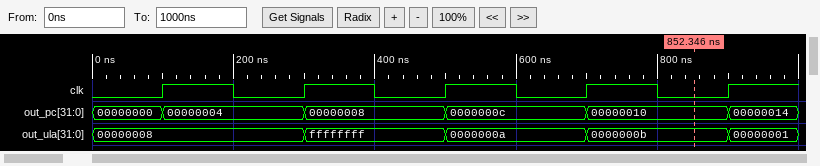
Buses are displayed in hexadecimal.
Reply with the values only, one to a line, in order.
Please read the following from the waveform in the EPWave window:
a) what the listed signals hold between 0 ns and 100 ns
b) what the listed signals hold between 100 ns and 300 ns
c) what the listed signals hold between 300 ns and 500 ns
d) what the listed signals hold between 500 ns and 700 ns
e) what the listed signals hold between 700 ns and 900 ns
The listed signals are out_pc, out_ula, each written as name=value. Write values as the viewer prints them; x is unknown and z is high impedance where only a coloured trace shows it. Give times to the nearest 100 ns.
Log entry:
out_pc=00000000, out_ula=00000008
out_pc=00000004, out_ula=00000008
out_pc=00000008, out_ula=ffffffff
out_pc=0000000c, out_ula=0000000a
out_pc=00000010, out_ula=0000000b
